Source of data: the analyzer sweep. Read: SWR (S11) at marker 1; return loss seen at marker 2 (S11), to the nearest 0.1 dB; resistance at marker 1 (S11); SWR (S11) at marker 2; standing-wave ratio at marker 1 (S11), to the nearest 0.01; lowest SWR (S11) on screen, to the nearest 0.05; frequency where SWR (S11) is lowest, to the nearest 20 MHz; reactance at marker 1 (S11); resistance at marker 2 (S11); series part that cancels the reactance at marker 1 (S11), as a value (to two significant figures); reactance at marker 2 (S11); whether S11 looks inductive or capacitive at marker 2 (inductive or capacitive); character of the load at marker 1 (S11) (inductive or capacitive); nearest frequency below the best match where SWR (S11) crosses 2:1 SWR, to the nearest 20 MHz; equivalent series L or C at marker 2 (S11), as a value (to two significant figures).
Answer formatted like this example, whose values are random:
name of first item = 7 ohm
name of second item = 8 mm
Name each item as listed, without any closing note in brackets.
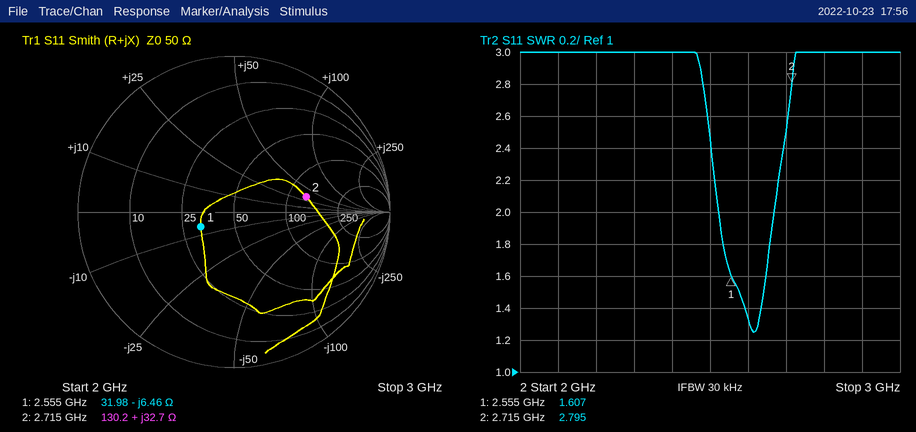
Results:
SWR (S11) at marker 1 = 1.607
return loss seen at marker 2 (S11), to the nearest 0.1 dB = 6.5 dB
resistance at marker 1 = 31.98 Ω
SWR (S11) at marker 2 = 2.795
standing-wave ratio at marker 1 (S11), to the nearest 0.01 = 1.61
lowest SWR (S11) on screen, to the nearest 0.05 = 1.25
frequency where SWR (S11) is lowest, to the nearest 20 MHz = 2.62 GHz
reactance at marker 1 = -6.46 Ω
resistance at marker 2 = 130.2 Ω
series part that cancels the reactance at marker 1 (S11), as a value = 400 pH
reactance at marker 2 = +32.7 Ω
whether S11 looks inductive or capacitive at marker 2 = inductive
character of the load at marker 1 (S11) = capacitive
nearest frequency below the best match where SWR (S11) crosses 2:1 SWR, to the nearest 20 MHz = 2.52 GHz
equivalent series L or C at marker 2 (S11), as a value = 1.9 nH
